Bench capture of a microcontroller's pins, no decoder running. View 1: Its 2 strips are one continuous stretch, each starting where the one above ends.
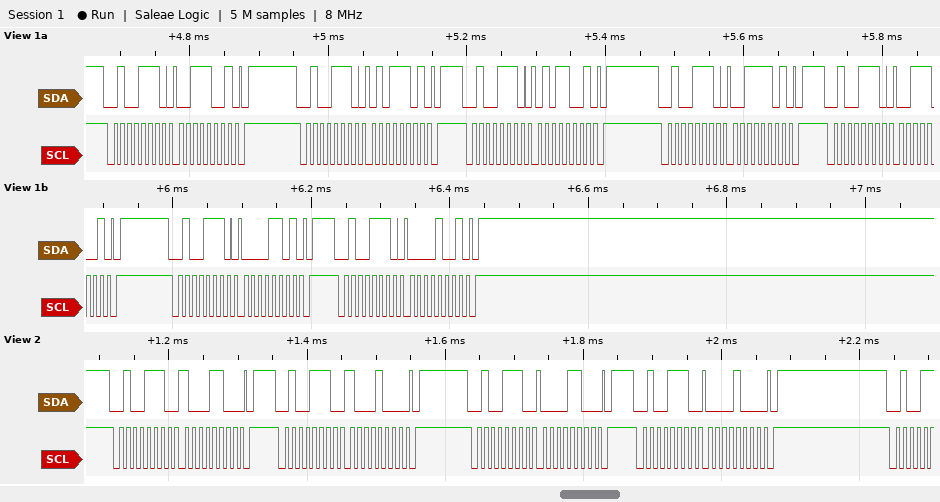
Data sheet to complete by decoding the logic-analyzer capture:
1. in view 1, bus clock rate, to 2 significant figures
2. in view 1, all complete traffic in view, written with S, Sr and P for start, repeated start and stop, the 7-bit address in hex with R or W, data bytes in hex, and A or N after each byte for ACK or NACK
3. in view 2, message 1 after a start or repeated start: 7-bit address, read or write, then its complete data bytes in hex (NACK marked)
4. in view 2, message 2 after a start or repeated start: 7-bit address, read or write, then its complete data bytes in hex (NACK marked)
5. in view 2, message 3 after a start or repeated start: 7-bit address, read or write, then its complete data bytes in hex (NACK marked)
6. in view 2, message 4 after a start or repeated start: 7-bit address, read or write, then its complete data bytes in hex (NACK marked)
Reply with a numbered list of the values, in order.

1. 100 kHz
2. S 27W A 39 A P S 27W A 5D A P S 27W A 59 A P S 27W A 3D A P S 27W A 39 A P S 27W A 0D A P S 27W A 09 A P
3. 0x27 write: 8C
4. 0x27 write: 88
5. 0x27 write: 0C
6. 0x27 write: 08
